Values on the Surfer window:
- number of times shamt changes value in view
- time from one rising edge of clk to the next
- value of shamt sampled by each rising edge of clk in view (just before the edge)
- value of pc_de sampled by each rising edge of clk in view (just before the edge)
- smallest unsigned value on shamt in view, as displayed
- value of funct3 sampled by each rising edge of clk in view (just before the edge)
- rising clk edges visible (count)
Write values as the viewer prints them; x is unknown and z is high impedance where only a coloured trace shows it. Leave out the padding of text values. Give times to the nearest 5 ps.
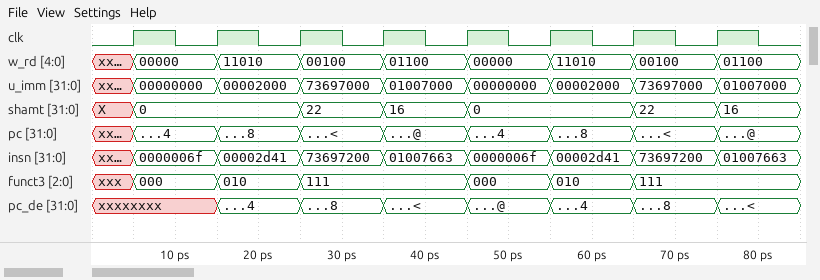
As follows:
6
10 ps
X, 0, 0, 22, 16, 0, 0, 22
xxxxxxxx, xxxxxxxx, 4, 8, <, @, 4, 8
0
xxx, 000, 010, 111, 111, 000, 010, 111
8
